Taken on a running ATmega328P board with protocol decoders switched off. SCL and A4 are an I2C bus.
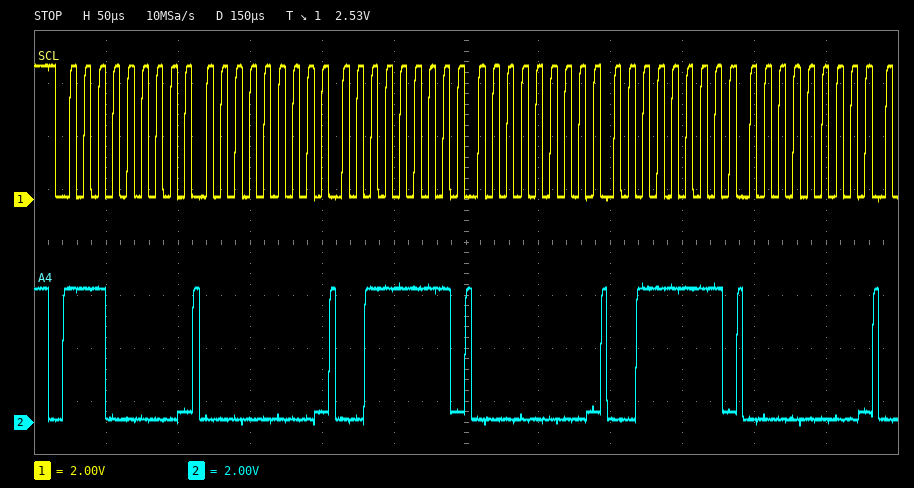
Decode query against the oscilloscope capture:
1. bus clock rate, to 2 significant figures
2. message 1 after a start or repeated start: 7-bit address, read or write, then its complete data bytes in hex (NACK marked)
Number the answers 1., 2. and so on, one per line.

1. 100 kHz
2. 0x70 write: 00 3F 00 3F 00
